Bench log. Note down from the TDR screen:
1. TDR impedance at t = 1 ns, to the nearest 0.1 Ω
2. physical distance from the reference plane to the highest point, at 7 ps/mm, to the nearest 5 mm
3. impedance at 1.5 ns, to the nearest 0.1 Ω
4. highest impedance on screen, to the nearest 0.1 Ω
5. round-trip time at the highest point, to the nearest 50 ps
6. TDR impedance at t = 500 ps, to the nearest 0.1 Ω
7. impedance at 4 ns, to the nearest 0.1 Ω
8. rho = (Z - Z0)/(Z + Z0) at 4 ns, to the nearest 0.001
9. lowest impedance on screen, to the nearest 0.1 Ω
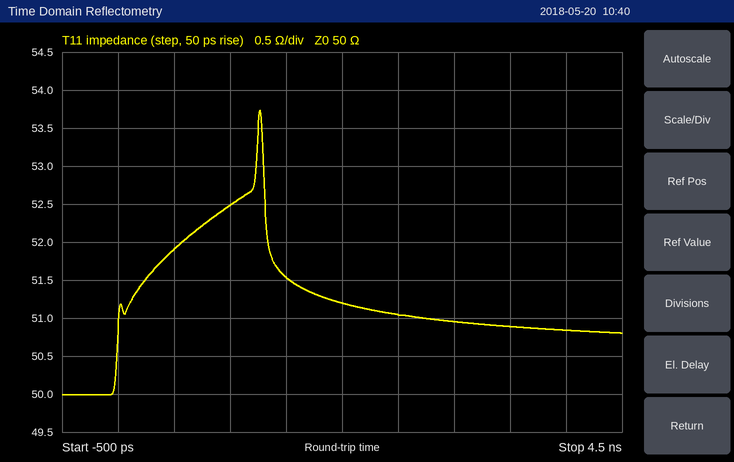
52.5 Ω
90 mm
51.5 Ω
53.7 Ω
1.25 ns
51.9 Ω
50.8 Ω
+0.008
50.0 Ω
